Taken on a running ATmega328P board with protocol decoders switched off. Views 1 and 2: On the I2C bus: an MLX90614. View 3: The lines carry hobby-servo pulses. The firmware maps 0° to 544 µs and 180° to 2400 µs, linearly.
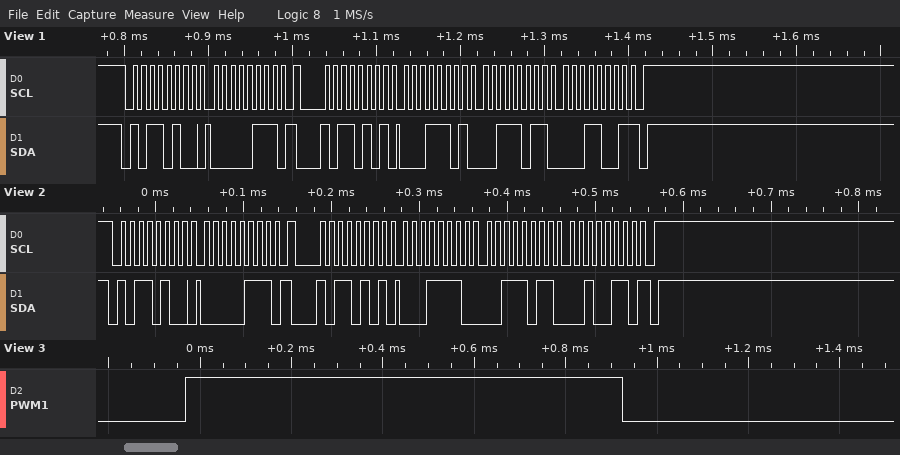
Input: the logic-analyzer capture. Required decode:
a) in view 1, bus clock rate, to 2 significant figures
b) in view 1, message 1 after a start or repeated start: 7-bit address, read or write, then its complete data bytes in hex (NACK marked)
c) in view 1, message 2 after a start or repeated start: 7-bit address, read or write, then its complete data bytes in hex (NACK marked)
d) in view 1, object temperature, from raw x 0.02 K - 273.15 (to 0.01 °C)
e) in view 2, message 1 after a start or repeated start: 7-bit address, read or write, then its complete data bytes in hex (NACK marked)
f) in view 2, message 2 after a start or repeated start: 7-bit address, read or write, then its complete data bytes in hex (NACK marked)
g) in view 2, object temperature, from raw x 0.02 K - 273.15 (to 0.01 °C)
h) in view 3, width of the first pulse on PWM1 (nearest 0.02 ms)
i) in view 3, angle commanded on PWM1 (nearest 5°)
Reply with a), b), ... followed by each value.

a) 100 kHz
b) 0x5A write: 07
c) 0x5A read: 1D 3B 19 NACK
d) 29.51 °C
e) 0x5A write: 07
f) 0x5A read: 1E 3B 26 NACK
g) 29.53 °C
h) 0.96 ms
i) 40°
